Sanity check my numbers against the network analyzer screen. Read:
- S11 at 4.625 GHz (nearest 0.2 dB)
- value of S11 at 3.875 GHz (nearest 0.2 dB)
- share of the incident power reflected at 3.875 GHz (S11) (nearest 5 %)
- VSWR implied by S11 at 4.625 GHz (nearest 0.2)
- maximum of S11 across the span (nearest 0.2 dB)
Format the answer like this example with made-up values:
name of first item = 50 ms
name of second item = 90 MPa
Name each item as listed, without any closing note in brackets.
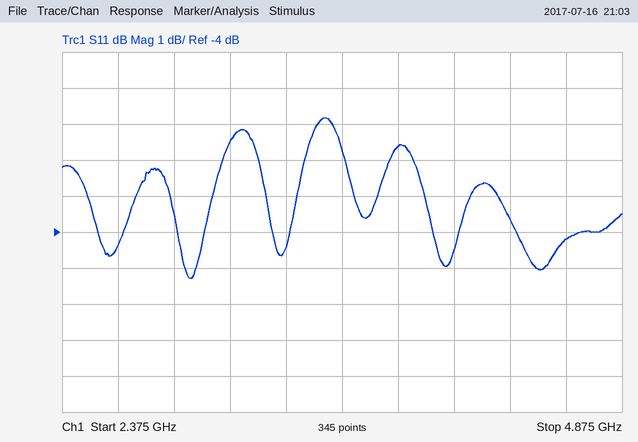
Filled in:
S11 at 4.625 GHz = -4.2 dB
value of S11 at 3.875 GHz = -1.6 dB
share of the incident power reflected at 3.875 GHz (S11) = 70 %
VSWR implied by S11 at 4.625 GHz = 4.2
maximum of S11 across the span = -0.8 dB
